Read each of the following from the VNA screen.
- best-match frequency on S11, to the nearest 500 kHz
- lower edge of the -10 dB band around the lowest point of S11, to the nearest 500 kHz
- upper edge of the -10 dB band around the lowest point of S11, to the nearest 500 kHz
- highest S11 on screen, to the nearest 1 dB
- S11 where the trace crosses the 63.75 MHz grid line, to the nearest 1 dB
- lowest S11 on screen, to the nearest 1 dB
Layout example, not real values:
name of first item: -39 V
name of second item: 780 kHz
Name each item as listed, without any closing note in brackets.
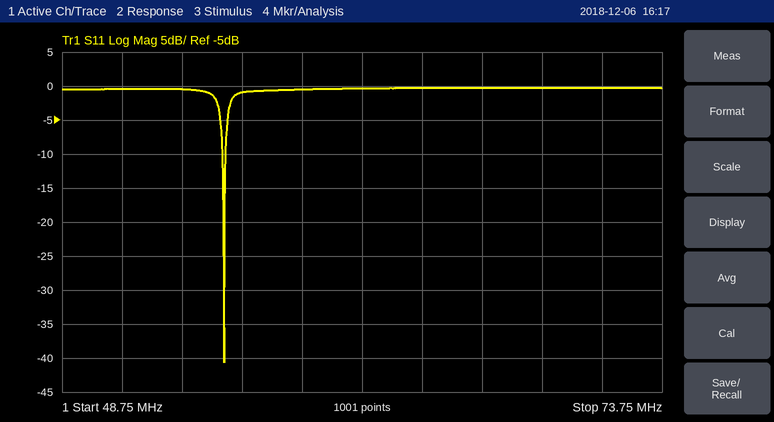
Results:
best-match frequency on S11, to the nearest 500 kHz: 55.5 MHz
lower edge of the -10 dB band around the lowest point of S11, to the nearest 500 kHz: 55.5 MHz
upper edge of the -10 dB band around the lowest point of S11, to the nearest 500 kHz: 55.5 MHz
highest S11 on screen, to the nearest 1 dB: 0 dB
S11 where the trace crosses the 63.75 MHz grid line, to the nearest 1 dB: 0 dB
lowest S11 on screen, to the nearest 1 dB: -41 dB
